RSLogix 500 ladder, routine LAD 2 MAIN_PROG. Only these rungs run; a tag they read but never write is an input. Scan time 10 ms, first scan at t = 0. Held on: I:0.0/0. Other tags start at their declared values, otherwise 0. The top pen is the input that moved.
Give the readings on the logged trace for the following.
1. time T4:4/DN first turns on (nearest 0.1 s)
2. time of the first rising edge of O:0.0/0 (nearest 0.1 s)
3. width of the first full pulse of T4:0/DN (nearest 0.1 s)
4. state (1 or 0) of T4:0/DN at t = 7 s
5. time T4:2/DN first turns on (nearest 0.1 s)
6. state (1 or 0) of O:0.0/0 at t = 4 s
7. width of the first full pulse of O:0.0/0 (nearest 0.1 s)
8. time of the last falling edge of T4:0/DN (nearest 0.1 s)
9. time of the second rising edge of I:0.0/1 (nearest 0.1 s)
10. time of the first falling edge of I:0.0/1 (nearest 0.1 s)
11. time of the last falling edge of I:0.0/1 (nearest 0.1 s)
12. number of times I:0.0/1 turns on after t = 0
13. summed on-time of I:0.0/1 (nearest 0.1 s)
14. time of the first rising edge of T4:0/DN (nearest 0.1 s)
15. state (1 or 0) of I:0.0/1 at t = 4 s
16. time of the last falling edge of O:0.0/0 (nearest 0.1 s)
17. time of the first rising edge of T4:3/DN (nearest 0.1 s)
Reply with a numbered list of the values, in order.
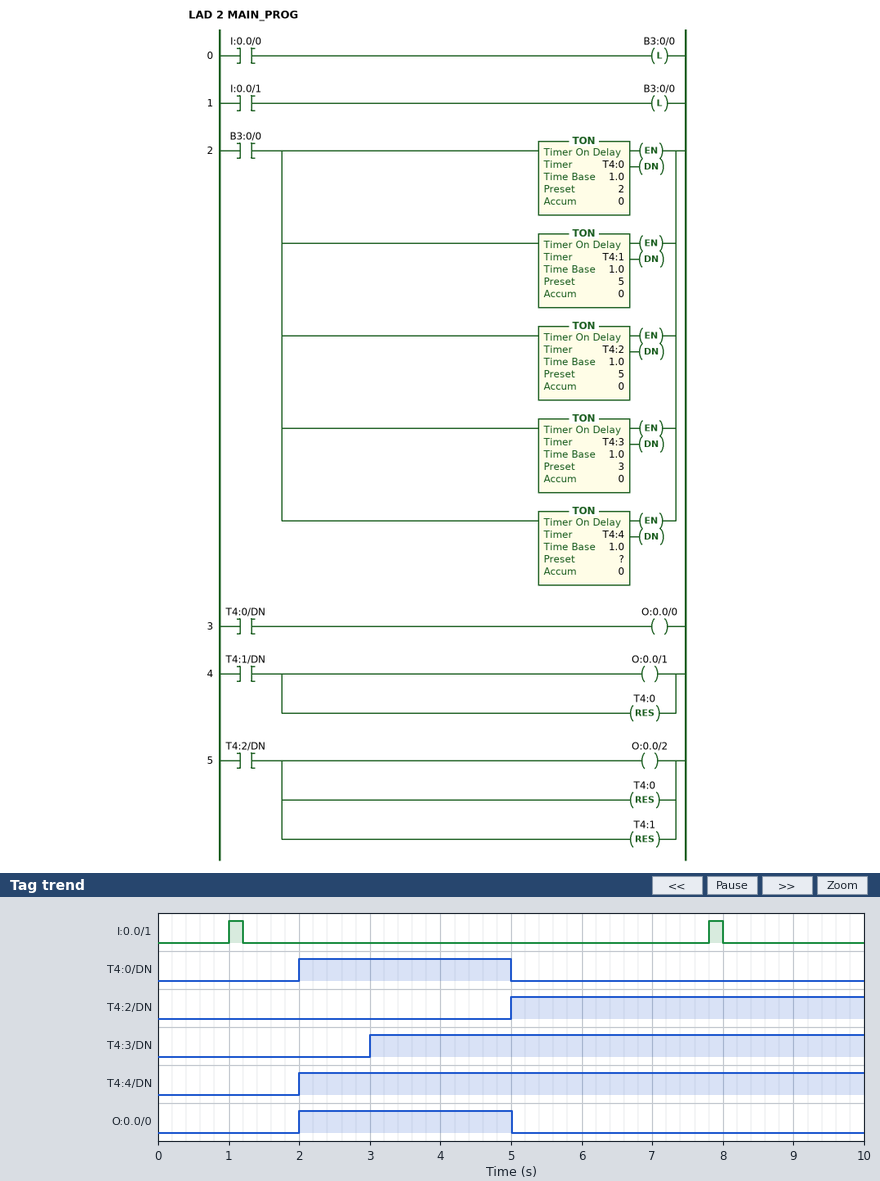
1. 2.0 s
2. 2.0 s
3. 3.0 s
4. 0
5. 5.0 s
6. 1
7. 3.0 s
8. 5.0 s
9. 7.8 s
10. 1.2 s
11. 8.0 s
12. 2
13. 0.4 s
14. 2.0 s
15. 0
16. 5.0 s
17. 3.0 s
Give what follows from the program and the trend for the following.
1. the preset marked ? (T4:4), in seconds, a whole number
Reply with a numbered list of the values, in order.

1. 2 s
